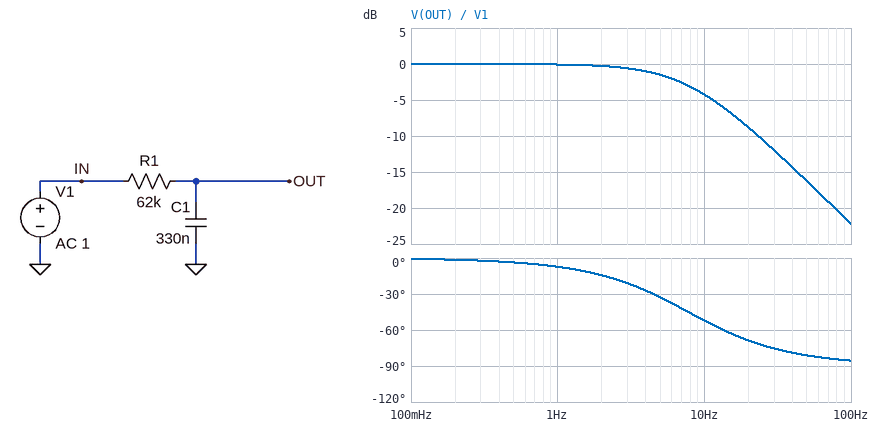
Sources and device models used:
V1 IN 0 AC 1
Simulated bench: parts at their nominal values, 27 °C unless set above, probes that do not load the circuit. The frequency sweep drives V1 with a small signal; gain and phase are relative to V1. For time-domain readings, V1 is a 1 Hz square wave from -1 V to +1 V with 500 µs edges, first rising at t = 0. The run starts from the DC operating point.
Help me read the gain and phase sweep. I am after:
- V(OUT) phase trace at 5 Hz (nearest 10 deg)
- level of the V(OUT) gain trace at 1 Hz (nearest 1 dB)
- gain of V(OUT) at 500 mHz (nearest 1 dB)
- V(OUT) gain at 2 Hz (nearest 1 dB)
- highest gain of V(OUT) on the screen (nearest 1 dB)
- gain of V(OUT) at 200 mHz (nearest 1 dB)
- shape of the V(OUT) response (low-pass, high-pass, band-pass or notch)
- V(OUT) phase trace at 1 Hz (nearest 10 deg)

-30 deg
0 dB
0 dB
0 dB
0 dB
0 dB
low-pass
-10 deg
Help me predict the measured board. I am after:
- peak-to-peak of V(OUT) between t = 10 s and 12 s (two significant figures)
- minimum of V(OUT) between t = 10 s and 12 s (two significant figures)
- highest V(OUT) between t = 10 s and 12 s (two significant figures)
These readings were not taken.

2.0 V
-1.0 V
1.0 V
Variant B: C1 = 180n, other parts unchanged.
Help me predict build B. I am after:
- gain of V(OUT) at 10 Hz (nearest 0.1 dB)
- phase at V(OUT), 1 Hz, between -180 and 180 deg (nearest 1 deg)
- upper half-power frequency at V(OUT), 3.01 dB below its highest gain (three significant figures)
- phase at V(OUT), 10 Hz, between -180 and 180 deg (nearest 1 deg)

-1.7 dB
-4 deg
14.3 Hz
-35 deg
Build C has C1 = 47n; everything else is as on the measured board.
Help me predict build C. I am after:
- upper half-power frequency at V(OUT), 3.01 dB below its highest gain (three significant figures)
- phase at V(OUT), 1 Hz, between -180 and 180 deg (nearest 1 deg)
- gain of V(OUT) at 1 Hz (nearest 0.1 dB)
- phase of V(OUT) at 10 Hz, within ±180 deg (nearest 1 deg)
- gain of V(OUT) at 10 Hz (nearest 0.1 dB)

54.6 Hz
-1 deg
0 dB
-10 deg
-0.1 dB
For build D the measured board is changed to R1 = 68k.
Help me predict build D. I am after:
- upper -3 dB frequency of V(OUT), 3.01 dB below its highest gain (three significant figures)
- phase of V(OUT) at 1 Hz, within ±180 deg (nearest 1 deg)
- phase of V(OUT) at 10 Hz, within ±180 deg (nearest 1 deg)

7.09 Hz
-8 deg
-55 deg
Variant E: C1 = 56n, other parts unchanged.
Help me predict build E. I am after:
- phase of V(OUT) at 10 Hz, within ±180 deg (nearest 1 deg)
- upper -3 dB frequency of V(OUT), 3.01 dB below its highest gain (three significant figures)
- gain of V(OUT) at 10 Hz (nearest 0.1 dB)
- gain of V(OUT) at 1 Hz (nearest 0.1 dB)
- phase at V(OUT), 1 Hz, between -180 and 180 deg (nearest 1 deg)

-12 deg
45.8 Hz
-0.2 dB
0 dB
-1 deg
